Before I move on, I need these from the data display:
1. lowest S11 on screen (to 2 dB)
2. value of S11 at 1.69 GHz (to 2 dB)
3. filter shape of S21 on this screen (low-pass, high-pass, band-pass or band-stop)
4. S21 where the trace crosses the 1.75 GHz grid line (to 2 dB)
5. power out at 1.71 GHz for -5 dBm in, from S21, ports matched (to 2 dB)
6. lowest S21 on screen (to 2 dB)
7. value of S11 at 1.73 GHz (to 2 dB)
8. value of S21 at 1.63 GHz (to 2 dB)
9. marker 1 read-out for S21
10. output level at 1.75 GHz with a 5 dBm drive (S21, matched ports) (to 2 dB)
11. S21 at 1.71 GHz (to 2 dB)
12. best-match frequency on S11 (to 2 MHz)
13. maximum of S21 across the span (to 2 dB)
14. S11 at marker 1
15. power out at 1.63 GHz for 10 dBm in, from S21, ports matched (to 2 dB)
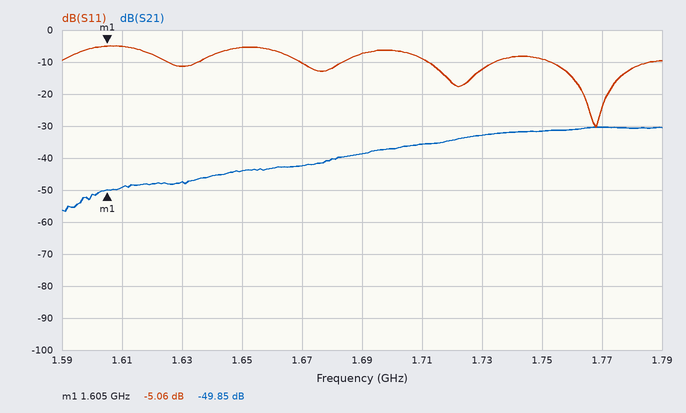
-30 dB
-8 dB
high-pass
-32 dB
-40 dBm
-56 dB
-12 dB
-48 dB
-49.85 dB
-26 dBm
-36 dB
1.768 GHz
-30 dB
-5.06 dB
-38 dBm
